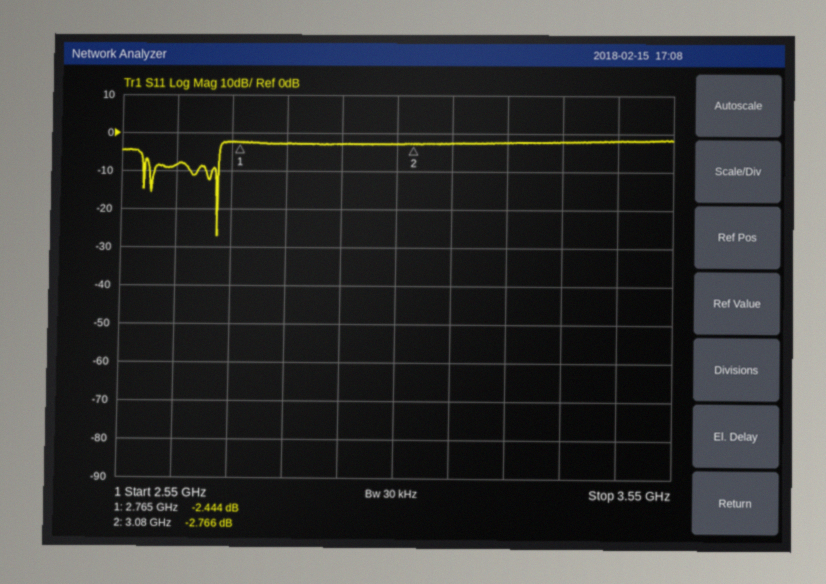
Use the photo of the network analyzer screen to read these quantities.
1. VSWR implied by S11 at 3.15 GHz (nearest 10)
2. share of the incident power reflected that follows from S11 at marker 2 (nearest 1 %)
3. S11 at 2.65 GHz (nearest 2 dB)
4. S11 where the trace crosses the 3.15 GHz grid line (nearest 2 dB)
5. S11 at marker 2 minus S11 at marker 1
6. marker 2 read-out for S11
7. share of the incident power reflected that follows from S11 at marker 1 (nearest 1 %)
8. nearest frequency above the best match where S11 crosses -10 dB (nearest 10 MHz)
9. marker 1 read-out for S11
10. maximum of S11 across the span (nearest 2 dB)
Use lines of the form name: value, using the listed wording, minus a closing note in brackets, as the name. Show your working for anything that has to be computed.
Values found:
VSWR implied by S11 at 3.15 GHz: |Γ| = 10^(-2/20) = 0.7943; VSWR = (1 + 0.7943)/(1 − 0.7943) ≈ 8.72, so 10 to the nearest 10
share of the incident power reflected that follows from S11 at marker 2: 10^(-2.766/10) ≈ 53 %
S11 at 2.65 GHz: -8 dB
S11 where the trace crosses the 3.15 GHz grid line: -2 dB
S11 at marker 2 minus S11 at marker 1: -2.766 − (-2.444) = -0.322 dB
marker 2 read-out for S11: -2.766 dB
share of the incident power reflected that follows from S11 at marker 1: 10^(-2.444/10) ≈ 57 %
nearest frequency above the best match where S11 crosses -10 dB: 2.73 GHz
marker 1 read-out for S11: -2.444 dB
maximum of S11 across the span: -2 dB
